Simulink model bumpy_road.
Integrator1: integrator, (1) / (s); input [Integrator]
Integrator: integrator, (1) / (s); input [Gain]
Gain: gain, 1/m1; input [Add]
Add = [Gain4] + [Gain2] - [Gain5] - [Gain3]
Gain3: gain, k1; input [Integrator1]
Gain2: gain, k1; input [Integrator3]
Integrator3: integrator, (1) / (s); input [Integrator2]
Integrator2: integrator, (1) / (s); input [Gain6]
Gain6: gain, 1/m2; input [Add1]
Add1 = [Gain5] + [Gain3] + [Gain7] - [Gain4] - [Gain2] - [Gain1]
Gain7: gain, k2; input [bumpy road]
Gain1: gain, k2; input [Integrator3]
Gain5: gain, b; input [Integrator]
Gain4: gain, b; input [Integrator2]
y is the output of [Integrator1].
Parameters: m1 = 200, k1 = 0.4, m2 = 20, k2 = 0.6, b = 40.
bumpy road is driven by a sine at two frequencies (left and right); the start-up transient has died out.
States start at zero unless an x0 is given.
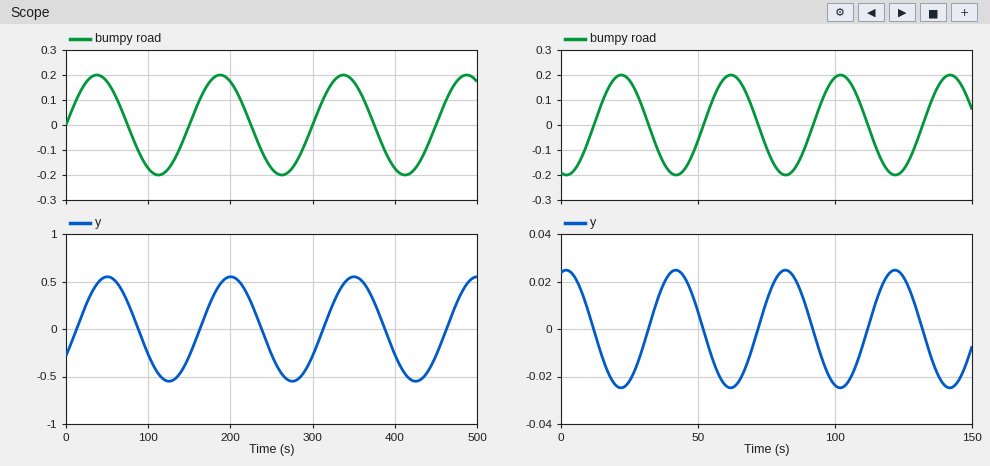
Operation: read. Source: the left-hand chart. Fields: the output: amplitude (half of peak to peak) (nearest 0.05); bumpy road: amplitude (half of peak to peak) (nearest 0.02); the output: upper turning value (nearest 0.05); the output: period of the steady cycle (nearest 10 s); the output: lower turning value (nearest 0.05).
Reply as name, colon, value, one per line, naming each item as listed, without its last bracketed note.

the output: amplitude (half of peak to peak): 0.55
bumpy road: amplitude (half of peak to peak): 0.20
the output: upper turning value: 0.55
the output: period of the steady cycle: 150 s
the output: lower turning value: -0.55
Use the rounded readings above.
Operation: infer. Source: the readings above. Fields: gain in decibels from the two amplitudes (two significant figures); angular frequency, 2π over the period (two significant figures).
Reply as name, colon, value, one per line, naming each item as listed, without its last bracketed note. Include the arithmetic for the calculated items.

gain in decibels from the two amplitudes: 20 log10(0.55 / 0.2) = 8.8 dB
angular frequency, 2π over the period: 2π / 150 = 0.042 rad/s
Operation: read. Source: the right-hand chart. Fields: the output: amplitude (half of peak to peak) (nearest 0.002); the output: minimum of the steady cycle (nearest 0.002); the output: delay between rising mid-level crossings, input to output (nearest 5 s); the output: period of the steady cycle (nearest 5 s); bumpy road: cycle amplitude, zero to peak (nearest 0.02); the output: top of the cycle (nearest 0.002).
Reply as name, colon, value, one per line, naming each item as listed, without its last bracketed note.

the output: amplitude (half of peak to peak): 0.024
the output: minimum of the steady cycle: -0.024
the output: delay between rising mid-level crossings, input to output: 20 s
the output: period of the steady cycle: 40 s
bumpy road: cycle amplitude, zero to peak: 0.20
the output: top of the cycle: 0.024
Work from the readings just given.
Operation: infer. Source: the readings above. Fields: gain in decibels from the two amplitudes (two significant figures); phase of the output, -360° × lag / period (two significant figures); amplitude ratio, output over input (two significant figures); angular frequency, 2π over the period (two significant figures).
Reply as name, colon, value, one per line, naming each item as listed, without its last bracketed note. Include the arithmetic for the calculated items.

gain in decibels from the two amplitudes: 20 log10(0.024 / 0.2) = -18 dB
phase of the output, -360° × lag / period: -360 × 20 / 40 = -180°
amplitude ratio, output over input: 0.024 / 0.2 = 0.12
angular frequency, 2π over the period: 2π / 40 = 0.16 rad/s
